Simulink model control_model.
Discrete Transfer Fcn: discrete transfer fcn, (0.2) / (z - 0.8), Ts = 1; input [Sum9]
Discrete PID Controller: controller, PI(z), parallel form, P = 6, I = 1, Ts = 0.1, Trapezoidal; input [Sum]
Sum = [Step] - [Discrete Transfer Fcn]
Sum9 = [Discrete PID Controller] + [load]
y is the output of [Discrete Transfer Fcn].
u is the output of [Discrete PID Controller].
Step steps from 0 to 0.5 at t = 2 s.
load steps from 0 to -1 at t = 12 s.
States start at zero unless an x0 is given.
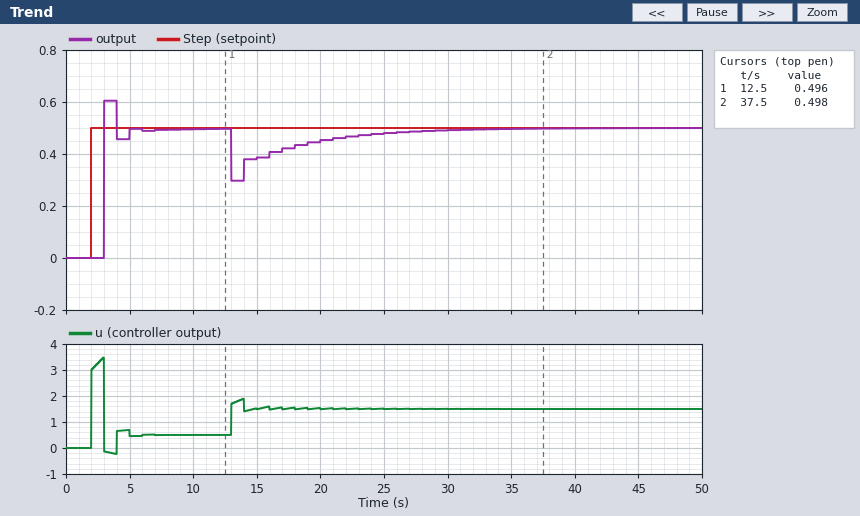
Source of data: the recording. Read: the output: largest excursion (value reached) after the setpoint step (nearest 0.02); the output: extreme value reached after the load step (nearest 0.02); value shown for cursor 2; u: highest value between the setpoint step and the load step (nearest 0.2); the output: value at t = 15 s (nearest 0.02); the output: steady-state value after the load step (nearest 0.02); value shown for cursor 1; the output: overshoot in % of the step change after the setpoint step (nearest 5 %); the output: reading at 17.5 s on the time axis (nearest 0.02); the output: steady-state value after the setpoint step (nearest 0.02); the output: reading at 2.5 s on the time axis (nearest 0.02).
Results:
0.60
0.30
0.498
3.4
0.38
0.50
0.496
20 %
0.42
0.50
0.00
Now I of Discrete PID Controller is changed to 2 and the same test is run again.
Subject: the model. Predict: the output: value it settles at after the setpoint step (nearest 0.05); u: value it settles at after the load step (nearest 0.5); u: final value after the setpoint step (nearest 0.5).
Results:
0.50
1.5
0.5
